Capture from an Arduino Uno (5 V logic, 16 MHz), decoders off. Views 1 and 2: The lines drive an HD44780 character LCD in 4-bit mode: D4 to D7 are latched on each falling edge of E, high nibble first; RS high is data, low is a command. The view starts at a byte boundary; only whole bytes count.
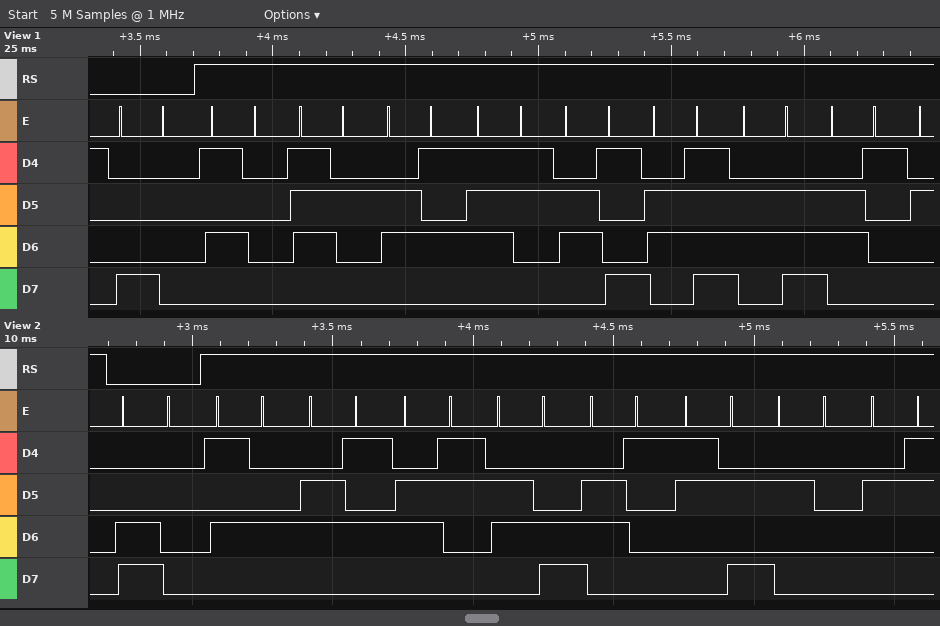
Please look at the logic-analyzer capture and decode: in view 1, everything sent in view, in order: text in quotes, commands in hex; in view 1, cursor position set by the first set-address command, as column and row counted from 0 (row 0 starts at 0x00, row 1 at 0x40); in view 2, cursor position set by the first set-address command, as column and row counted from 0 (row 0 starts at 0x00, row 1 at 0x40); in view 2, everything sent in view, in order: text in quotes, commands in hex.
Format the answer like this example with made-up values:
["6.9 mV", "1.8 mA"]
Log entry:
["0x80 \"Presiona\"", "column 0, row 0", "column 0, row 1", "0xC0 \"Tecla: #\""]
